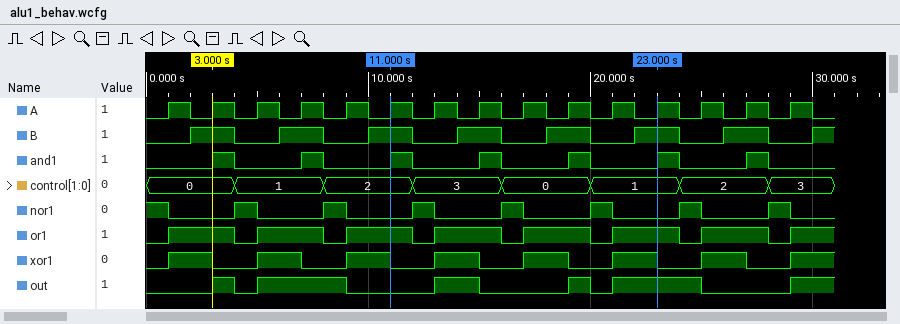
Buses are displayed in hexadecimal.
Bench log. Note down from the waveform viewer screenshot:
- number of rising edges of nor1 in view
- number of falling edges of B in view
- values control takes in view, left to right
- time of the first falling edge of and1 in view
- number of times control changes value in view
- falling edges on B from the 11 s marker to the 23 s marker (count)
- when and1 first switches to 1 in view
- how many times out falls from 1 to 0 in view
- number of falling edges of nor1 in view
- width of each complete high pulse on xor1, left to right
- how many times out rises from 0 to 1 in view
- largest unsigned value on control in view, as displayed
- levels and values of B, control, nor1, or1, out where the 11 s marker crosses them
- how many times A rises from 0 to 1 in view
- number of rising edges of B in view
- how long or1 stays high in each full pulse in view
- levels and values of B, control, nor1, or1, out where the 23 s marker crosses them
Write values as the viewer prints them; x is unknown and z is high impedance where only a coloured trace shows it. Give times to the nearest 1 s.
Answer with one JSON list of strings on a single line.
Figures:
["7", "7", "0, 1, 2, 3, 0, 1, 2, 3", "4 s", "7", "3", "3 s", "5", "8", "2 s, 2 s, 2 s, 2 s, 2 s, 2 s, 2 s", "6", "3", "B=1, control=2, nor1=0, or1=1, out=0", "15", "8", "3 s, 3 s, 3 s, 3 s, 3 s, 3 s, 3 s", "B=1, control=1, nor1=0, or1=1, out=1"]
